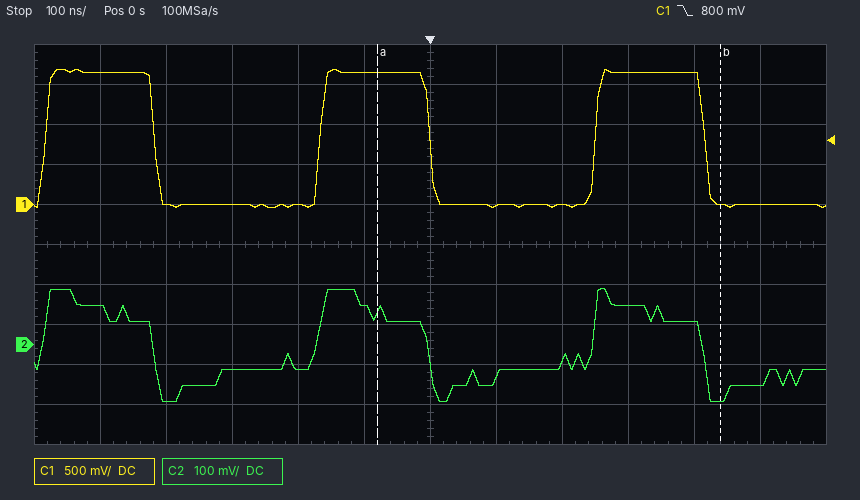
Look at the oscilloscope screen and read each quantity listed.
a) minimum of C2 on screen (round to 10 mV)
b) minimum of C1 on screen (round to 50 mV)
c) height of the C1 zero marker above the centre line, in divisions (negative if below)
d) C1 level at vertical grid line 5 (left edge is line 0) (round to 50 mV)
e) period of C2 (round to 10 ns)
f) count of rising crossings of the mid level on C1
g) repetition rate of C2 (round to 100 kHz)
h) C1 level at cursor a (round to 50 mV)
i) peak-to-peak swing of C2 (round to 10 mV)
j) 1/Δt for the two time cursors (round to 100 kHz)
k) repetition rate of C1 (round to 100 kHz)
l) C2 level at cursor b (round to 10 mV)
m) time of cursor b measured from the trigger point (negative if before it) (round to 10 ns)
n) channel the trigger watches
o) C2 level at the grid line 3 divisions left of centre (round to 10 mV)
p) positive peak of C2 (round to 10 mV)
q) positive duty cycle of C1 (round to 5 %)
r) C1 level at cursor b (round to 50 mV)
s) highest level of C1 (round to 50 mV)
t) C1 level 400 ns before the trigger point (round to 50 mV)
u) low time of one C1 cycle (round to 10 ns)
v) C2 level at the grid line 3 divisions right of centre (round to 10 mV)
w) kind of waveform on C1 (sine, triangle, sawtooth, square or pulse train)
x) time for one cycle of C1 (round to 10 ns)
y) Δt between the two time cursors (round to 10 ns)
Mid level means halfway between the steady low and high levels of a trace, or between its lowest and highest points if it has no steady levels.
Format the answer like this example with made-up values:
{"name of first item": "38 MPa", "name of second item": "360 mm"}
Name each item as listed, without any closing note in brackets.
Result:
{"minimum of C2 on screen": "-140 mV", "minimum of C1 on screen": "-50 mV", "height of the C1 zero marker above the centre line, in divisions": "+1.0 div", "C1 level at vertical grid line 5 (left edge is line 0)": "1.65 V", "period of C2": "420 ns", "count of rising crossings of the mid level on C1": "3", "repetition rate of C2": "2.4 MHz", "C1 level at cursor a": "1.65 V", "peak-to-peak swing of C2": "280 mV", "1/Δt for the two time cursors": "1.9 MHz", "repetition rate of C1": "2.4 MHz", "C2 level at cursor b": "-140 mV", "time of cursor b measured from the trigger point (negative if before it)": "+440 ns", "channel the trigger watches": "C1", "C2 level at the grid line 3 divisions left of centre": "-60 mV", "positive peak of C2": "140 mV", "positive duty cycle of C1": "40 %", "C1 level at cursor b": "0 mV", "highest level of C1": "1.70 V", "C1 level 400 ns before the trigger point": "0 mV", "low time of one C1 cycle": "250 ns", "C2 level at the grid line 3 divisions right of centre": "100 mV", "kind of waveform on C1": "pulse train", "time for one cycle of C1": "420 ns", "Δt between the two time cursors": "520 ns"}
